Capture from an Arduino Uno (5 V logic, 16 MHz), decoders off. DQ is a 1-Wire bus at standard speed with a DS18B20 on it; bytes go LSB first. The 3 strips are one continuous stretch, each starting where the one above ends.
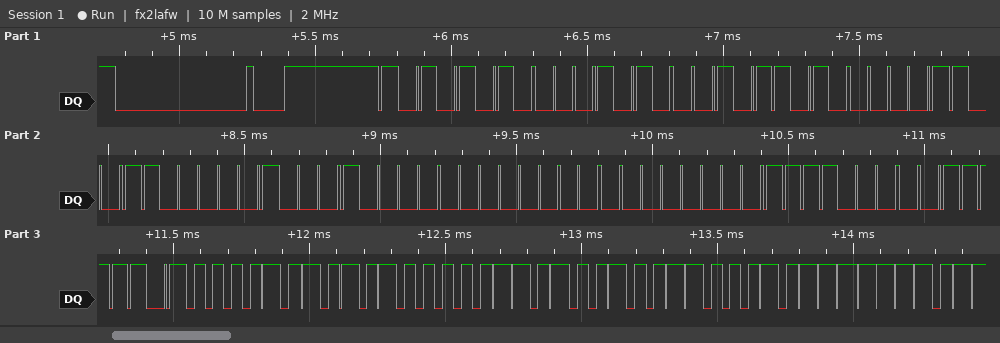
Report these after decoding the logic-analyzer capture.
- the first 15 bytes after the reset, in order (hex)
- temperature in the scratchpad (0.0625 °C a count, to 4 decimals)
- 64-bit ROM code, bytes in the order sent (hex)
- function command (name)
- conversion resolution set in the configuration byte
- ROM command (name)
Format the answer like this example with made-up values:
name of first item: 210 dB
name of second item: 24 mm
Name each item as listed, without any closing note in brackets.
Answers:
the first 15 bytes after the reset, in order: 55 28 5A 30 83 08 00 00 0F BE 50 05 4B 46 7F
temperature in the scratchpad: 85.0000 °C
64-bit ROM code, bytes in the order sent: 28 5A 30 83 08 00 00 0F
function command: Read Scratchpad
conversion resolution set in the configuration byte: 12 bits
ROM command: Match ROM
